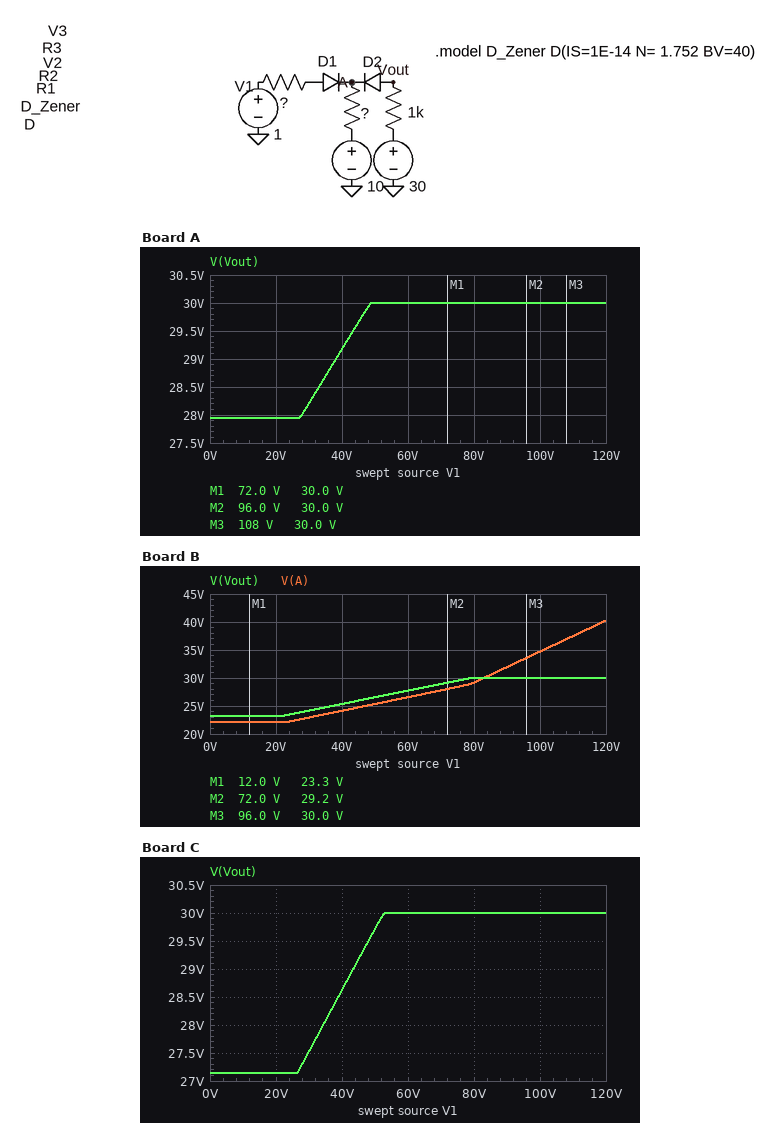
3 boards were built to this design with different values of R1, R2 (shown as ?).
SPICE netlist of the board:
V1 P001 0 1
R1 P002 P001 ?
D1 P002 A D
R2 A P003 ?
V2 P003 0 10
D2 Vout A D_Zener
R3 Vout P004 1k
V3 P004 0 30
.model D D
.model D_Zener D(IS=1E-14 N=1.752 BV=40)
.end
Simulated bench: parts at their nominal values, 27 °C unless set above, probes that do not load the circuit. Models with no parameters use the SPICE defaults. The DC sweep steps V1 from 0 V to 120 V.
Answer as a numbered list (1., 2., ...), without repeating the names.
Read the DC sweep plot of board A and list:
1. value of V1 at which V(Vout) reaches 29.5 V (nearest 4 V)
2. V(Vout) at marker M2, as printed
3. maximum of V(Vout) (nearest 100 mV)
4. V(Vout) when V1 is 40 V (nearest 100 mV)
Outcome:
1. 44 V
2. 30.0 V
3. 30.0 V
4. 29.2 V
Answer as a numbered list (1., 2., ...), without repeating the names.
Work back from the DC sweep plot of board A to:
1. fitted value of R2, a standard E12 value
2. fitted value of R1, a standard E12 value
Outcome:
1. 8.2 kΩ
2. 8.2 kΩ
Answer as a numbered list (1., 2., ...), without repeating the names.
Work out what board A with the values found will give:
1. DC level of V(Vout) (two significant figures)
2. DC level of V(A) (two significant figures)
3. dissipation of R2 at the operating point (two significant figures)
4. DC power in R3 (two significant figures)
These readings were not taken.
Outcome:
1. 28 V
2. 27 V
3. 34 mW
4. 4.2 mW
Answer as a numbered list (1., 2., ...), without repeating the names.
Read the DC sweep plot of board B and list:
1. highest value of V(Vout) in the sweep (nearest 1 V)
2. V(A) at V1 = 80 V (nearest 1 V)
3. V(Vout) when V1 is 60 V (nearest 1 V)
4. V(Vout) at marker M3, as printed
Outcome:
1. 30 V
2. 29 V
3. 28 V
4. 30.0 V
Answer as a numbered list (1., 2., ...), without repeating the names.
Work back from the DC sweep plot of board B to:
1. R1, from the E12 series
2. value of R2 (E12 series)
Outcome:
1. 4.7 kΩ
2. 1.8 kΩ
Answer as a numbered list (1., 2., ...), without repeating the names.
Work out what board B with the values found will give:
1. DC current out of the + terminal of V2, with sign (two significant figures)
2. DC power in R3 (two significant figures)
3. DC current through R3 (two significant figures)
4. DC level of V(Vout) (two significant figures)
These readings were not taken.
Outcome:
1. -6.7 mA
2. 45 mW
3. 6.7 mA
4. 23 V
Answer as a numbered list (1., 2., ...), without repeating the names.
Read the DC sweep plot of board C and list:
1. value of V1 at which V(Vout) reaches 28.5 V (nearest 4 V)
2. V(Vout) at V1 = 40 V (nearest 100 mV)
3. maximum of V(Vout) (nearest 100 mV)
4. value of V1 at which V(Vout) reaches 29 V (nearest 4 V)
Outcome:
1. 40 V
2. 28.6 V
3. 30.0 V
4. 44 V
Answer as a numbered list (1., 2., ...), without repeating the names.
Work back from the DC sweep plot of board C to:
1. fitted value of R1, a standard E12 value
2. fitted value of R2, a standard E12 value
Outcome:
1. 6.8 kΩ
2. 5.6 kΩ
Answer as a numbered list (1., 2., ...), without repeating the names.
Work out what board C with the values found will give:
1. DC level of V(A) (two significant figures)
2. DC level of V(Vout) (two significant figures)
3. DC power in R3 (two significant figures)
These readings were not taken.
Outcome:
1. 26 V
2. 27 V
3. 8.1 mW
